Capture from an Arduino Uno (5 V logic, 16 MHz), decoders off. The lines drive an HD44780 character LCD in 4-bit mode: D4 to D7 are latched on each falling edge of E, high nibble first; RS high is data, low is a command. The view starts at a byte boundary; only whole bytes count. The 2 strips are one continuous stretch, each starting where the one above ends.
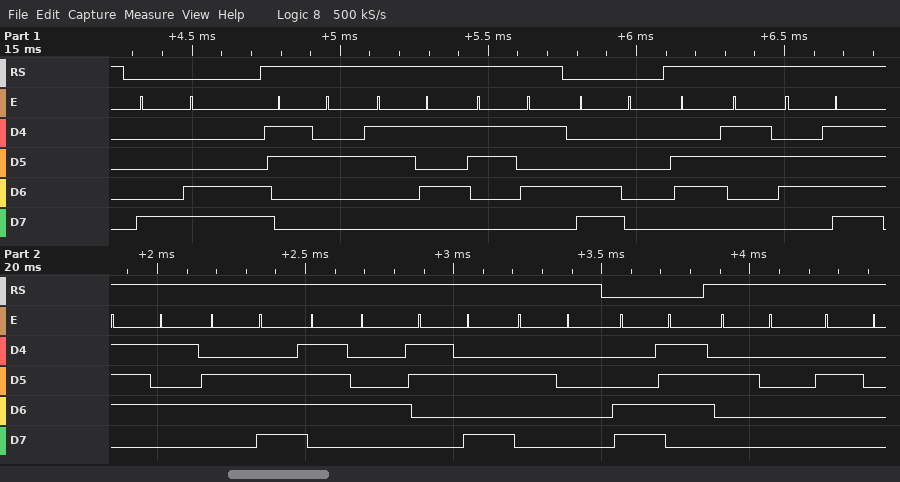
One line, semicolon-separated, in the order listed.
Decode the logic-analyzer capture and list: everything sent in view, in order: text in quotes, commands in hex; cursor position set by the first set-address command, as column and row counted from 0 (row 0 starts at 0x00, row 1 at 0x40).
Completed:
0x8C "255" 0xC0 "count: " 0xC7 "  "; column 12, row 0
